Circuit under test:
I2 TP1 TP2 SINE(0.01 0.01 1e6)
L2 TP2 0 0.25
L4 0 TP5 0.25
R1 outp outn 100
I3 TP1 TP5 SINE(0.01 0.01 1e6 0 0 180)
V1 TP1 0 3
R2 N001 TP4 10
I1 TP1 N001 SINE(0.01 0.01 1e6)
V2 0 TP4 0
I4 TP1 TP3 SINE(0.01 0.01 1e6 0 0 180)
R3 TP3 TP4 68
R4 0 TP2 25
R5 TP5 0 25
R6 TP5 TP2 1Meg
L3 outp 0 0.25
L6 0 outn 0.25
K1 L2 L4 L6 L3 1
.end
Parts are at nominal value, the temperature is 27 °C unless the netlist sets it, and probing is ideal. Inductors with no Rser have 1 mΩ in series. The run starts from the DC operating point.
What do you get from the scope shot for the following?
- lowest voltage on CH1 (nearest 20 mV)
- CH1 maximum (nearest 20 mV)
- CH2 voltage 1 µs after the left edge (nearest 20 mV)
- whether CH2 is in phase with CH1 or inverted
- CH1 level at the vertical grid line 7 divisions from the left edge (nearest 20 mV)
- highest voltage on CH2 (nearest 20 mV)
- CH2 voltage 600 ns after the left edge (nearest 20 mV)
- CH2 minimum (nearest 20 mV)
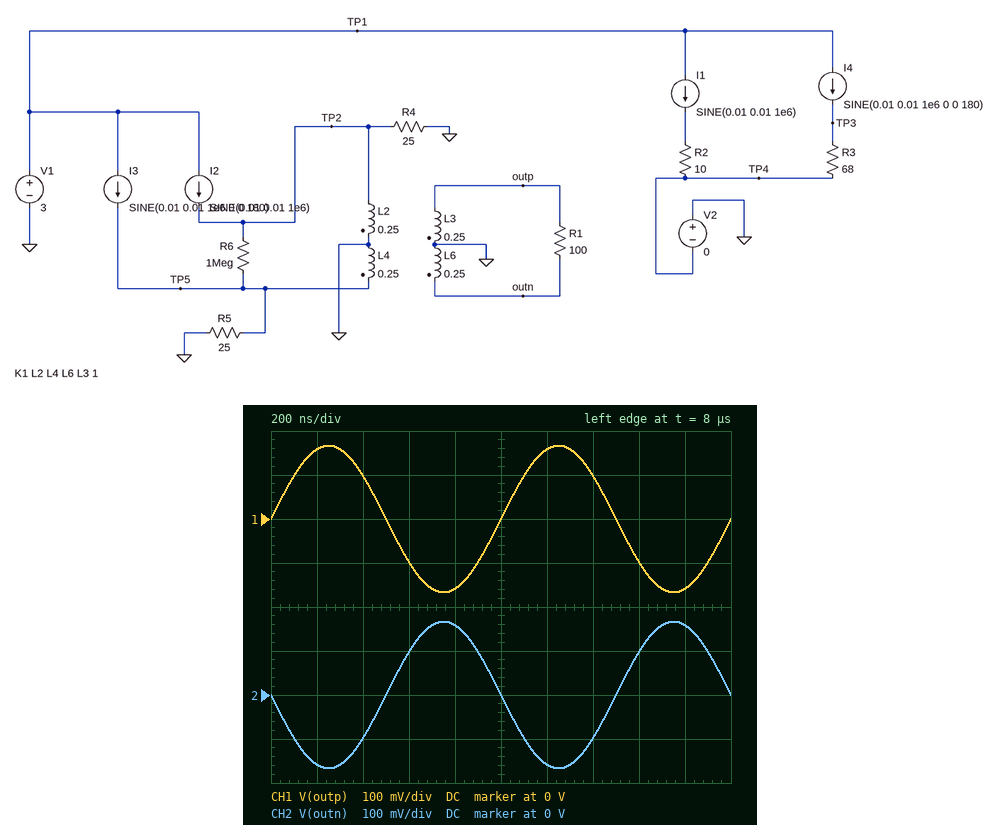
-160 mV
160 mV
0 V
inverted
100 mV
160 mV
100 mV
-160 mV
